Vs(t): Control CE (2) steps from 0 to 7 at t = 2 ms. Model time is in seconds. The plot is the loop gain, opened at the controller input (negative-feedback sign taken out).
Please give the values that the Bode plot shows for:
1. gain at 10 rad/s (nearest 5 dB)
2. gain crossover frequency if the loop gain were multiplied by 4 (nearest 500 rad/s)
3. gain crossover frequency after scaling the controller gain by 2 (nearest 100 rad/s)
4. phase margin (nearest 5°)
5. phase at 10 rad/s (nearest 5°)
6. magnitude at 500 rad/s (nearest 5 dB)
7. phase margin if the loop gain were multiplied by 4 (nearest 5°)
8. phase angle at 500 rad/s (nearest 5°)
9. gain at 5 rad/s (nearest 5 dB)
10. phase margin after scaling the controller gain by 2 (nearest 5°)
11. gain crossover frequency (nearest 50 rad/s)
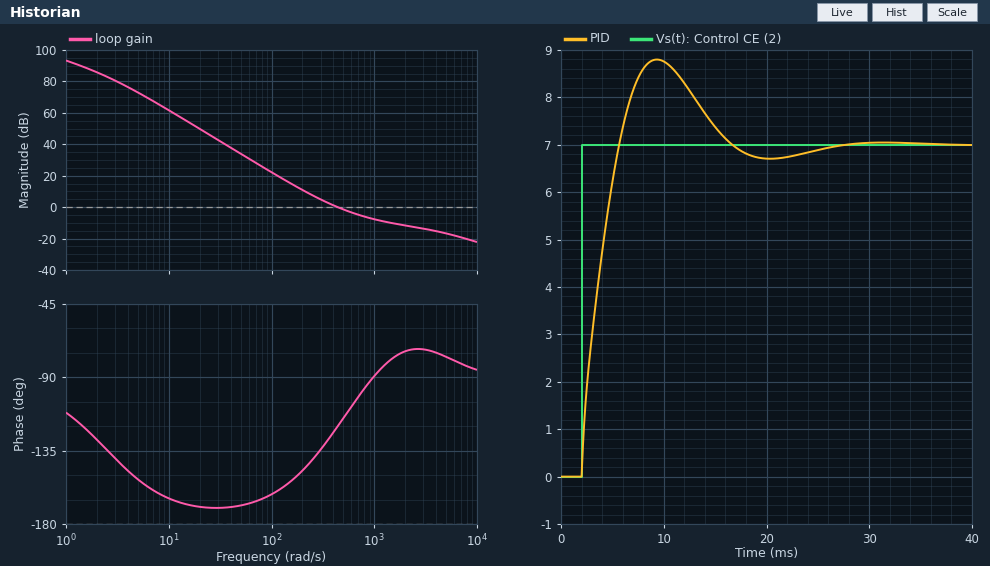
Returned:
60 dB
2000 rad/s
800 rad/s
60°
-165°
0 dB
105°
-115°
75 dB
85°
450 rad/s
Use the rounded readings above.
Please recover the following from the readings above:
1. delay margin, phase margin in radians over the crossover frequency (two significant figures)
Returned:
0.0023 s
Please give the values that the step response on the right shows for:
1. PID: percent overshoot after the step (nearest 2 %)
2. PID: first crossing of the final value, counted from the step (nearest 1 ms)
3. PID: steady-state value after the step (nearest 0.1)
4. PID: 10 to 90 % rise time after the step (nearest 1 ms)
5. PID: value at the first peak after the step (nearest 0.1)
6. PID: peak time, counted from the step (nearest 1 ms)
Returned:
26 %
4 ms
7.0
3 ms
8.8
7 ms
